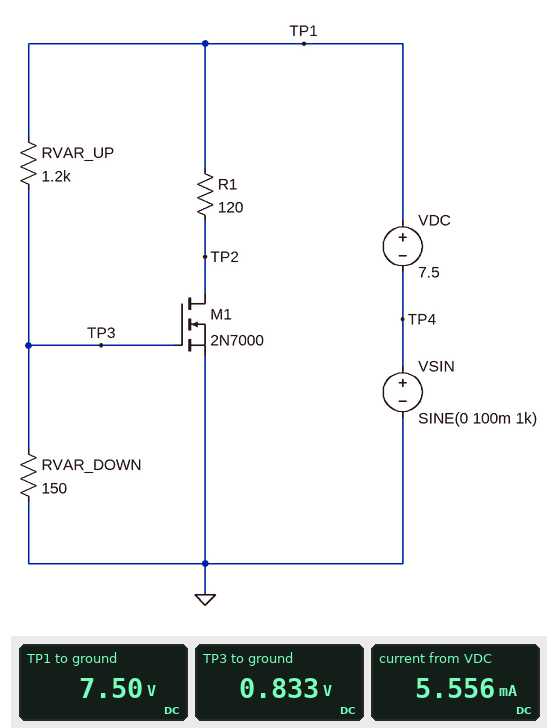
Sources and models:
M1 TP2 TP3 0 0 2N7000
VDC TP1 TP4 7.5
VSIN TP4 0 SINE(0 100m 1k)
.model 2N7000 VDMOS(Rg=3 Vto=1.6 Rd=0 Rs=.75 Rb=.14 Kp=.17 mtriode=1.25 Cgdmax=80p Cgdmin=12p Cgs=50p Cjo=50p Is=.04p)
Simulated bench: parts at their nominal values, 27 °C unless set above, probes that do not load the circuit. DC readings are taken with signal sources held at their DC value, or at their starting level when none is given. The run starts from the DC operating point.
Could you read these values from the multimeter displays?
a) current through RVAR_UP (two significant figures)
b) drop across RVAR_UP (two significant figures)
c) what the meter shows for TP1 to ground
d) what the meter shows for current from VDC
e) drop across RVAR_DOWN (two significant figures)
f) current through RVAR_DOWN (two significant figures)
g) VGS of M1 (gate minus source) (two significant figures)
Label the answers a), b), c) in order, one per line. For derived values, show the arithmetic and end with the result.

a) (7.5 V - 833 mV) / 1.2 kΩ = 5.6 mA
b) 7.5 V - 833 mV = 6.7 V
c) 7.50 V
d) 5.556 mA
e) 833 mV = 830 mV
f) (833 mV) / 150 Ω = 5.6 mA
g) 833 mV = 830 mV
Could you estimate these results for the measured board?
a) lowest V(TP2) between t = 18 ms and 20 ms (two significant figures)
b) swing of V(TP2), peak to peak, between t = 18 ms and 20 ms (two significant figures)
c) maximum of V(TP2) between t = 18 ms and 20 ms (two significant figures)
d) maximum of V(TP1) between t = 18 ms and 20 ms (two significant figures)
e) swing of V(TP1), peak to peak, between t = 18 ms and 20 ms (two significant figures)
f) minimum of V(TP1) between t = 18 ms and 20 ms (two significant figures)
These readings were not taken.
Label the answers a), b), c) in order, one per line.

a) 7.4 V
b) 200 mV
c) 7.6 V
d) 7.6 V
e) 200 mV
f) 7.4 V
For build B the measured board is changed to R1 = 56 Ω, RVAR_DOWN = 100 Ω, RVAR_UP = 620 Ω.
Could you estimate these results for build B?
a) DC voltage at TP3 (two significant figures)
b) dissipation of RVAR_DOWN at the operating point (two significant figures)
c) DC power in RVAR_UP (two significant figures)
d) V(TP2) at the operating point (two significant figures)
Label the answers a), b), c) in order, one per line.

a) 1.0 V
b) 11 mW
c) 67 mW
d) 7.5 V
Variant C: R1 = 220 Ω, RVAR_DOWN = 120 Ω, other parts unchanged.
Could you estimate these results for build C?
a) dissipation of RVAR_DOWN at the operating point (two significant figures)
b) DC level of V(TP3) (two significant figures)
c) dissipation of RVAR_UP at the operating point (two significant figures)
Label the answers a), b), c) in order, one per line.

a) 3.9 mW
b) 680 mV
c) 39 mW
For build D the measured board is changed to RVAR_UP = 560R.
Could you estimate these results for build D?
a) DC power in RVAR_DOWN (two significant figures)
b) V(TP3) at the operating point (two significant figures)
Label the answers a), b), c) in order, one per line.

a) 17 mW
b) 1.6 V
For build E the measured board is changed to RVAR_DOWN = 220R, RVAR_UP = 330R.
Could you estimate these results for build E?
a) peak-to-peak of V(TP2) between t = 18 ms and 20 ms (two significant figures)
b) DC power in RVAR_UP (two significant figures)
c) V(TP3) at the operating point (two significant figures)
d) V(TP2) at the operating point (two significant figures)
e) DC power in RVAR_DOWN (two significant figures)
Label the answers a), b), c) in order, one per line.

a) 8.4 mV
b) 61 mW
c) 3.0 V
d) 280 mV
e) 41 mW
